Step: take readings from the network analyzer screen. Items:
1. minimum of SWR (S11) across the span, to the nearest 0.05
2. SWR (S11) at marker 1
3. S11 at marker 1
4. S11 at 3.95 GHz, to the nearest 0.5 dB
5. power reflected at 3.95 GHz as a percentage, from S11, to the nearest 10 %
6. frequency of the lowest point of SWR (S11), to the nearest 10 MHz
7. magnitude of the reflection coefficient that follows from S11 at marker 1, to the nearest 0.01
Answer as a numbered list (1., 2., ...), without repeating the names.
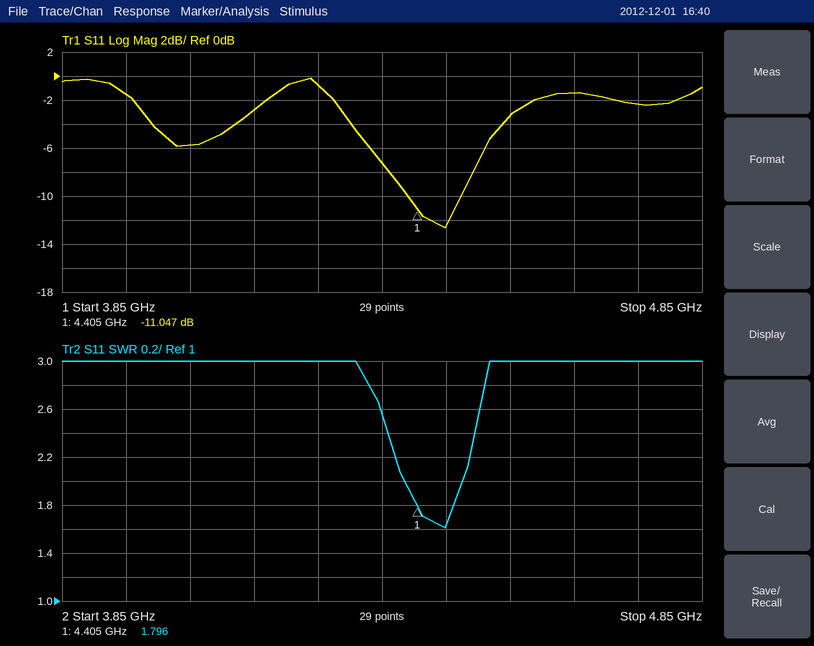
1. 1.60
2. 1.796
3. -11.047 dB
4. -1.5 dB
5. 70 %
6. 4.45 GHz
7. 0.28
